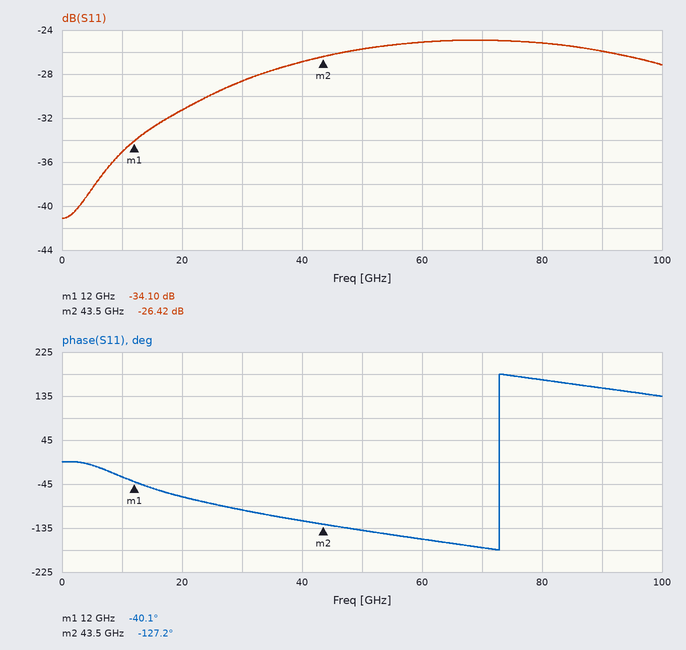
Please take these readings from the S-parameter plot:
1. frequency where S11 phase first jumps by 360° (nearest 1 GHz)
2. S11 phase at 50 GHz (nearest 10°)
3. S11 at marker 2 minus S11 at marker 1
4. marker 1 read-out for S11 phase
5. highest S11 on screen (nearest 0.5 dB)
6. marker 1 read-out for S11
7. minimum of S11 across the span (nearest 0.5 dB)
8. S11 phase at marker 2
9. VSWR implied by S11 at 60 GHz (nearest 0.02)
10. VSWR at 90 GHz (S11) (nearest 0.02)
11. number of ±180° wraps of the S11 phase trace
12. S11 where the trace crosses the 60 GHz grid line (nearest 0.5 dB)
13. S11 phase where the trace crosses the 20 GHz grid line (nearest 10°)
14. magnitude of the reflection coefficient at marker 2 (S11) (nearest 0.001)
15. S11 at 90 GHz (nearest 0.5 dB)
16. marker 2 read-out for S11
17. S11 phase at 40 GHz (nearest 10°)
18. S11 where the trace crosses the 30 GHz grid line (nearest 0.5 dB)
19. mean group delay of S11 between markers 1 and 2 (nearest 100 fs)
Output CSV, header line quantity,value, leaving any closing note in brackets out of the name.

quantity,value
frequency where S11 phase first jumps by 360°,73 GHz
S11 phase at 50 GHz,-140°
S11 at marker 2 minus S11 at marker 1,7.68 dB
marker 1 read-out for S11 phase,-40.1°
highest S11 on screen,-25.0 dB
marker 1 read-out for S11,-34.10 dB
minimum of S11 across the span,-41.0 dB
S11 phase at marker 2,-127.2°
VSWR implied by S11 at 60 GHz,1.12
VSWR at 90 GHz (S11),1.10
number of ±180° wraps of the S11 phase trace,1
S11 where the trace crosses the 60 GHz grid line,-25.0 dB
S11 phase where the trace crosses the 20 GHz grid line,-70°
magnitude of the reflection coefficient at marker 2 (S11),0.048
S11 at 90 GHz,-26.0 dB
marker 2 read-out for S11,-26.42 dB
S11 phase at 40 GHz,-120°
S11 where the trace crosses the 30 GHz grid line,-28.5 dB
mean group delay of S11 between markers 1 and 2,7.7 ps
